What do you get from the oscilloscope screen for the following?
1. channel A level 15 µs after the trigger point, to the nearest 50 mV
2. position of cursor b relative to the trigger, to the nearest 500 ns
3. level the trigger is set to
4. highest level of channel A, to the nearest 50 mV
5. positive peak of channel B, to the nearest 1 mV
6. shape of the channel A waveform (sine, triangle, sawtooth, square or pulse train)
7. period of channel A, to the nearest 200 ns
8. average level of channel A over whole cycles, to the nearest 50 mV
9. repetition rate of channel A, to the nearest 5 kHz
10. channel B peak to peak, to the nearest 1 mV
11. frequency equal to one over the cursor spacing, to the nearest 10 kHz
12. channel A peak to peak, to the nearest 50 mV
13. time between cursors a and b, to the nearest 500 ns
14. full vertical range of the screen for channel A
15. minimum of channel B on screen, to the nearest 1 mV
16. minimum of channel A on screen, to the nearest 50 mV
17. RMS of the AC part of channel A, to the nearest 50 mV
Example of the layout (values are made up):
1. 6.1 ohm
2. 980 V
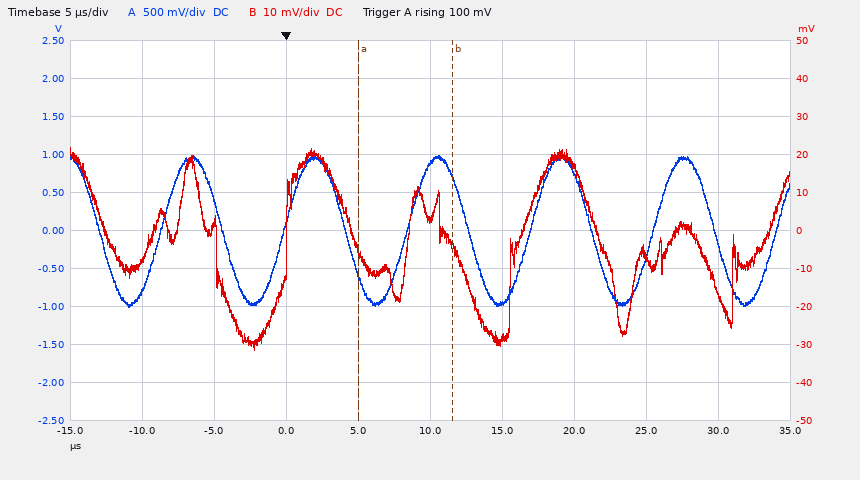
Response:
1. -950 mV
2. +11.5 µs
3. 100 mV
4. 1.00 V
5. 22 mV
6. sine
7. 8.6 µs
8. 0 mV
9. 115 kHz
10. 53 mV
11. 150 kHz
12. 2.00 V
13. 6.5 µs
14. 5 V
15. -31 mV
16. -1.00 V
17. 700 mV
